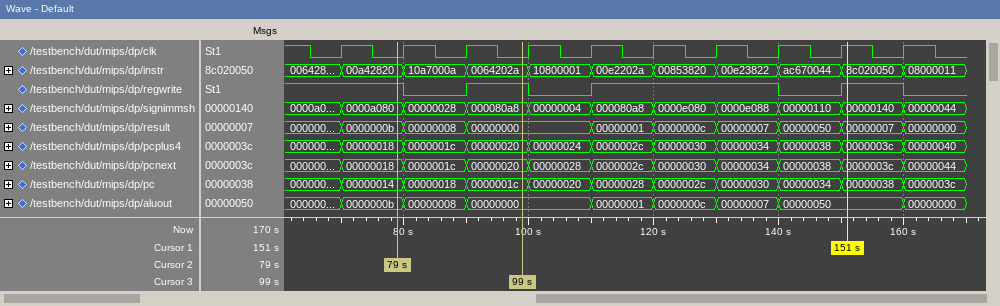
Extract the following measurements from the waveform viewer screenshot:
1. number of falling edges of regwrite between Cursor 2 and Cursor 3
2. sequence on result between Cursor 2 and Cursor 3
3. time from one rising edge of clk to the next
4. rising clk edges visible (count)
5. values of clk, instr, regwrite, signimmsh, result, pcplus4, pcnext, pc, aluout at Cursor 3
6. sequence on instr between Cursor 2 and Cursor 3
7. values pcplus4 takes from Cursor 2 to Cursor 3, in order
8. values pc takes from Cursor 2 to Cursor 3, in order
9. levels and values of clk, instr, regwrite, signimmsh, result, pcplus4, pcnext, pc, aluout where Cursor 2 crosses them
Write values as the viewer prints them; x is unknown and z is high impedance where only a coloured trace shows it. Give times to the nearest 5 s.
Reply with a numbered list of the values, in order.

1. 1
2. 0000000b, 00000008, 00000000
3. 10 s
4. 10
5. clk=0, instr=0064202a, regwrite=1, signimmsh=000080a8, result=00000000, pcplus4=00000020, pcnext=00000020, pc=0000001c, aluout=00000000
6. 00a42820, 10a7000a, 0064202a
7. 00000018, 0000001c, 00000020
8. 00000014, 00000018, 0000001c
9. clk=0, instr=00a42820, regwrite=1, signimmsh=0000a080, result=0000000b, pcplus4=00000018, pcnext=00000018, pc=00000014, aluout=0000000b
